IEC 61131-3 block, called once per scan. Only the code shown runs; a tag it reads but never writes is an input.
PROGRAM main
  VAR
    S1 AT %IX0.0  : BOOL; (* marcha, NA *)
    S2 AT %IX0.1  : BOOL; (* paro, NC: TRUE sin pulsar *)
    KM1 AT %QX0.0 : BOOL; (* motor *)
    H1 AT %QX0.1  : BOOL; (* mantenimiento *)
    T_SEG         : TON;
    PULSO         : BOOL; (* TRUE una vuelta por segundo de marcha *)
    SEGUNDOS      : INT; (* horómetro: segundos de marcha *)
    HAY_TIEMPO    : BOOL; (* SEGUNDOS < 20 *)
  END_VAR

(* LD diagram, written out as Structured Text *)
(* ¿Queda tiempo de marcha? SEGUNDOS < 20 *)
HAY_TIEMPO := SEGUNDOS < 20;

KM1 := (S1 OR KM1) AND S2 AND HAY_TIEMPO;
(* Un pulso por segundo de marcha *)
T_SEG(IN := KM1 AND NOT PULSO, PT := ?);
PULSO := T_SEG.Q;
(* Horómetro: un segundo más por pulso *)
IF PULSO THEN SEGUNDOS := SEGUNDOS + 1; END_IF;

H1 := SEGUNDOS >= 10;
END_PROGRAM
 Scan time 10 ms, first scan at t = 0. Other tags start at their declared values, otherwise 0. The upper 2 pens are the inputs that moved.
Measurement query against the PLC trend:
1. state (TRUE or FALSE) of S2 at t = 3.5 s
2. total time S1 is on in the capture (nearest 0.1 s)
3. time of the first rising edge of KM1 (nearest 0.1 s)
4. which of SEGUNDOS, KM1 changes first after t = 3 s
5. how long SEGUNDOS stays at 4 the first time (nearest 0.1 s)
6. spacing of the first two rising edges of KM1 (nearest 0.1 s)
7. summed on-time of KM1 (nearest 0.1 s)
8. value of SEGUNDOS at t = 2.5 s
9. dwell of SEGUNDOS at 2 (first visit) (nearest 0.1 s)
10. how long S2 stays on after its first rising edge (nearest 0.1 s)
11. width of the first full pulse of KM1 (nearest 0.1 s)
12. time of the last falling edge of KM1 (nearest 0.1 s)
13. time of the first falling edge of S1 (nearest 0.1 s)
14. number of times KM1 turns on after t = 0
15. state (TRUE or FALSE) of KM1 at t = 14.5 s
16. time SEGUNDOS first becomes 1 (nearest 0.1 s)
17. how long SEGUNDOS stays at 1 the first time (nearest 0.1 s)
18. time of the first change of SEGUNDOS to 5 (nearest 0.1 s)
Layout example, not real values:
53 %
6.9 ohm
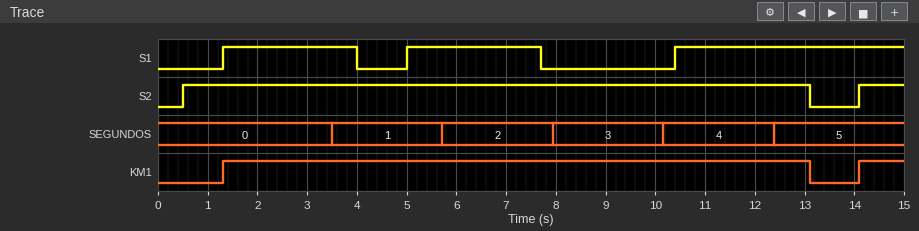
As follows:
TRUE
10.0 s
1.3 s
SEGUNDOS
2.2 s
12.8 s
12.7 s
0
2.2 s
12.6 s
11.8 s
13.1 s
4.0 s
2
TRUE
3.5 s
2.2 s
12.4 s
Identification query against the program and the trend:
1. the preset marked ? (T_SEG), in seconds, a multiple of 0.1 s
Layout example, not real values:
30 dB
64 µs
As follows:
2.2 s
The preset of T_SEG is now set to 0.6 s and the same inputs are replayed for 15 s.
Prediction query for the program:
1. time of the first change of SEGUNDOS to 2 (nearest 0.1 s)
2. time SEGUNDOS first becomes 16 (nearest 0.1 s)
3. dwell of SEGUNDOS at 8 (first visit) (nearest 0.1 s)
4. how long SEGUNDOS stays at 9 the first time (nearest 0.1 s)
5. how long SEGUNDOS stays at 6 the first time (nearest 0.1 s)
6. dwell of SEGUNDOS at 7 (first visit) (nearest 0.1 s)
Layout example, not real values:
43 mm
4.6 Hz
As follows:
2.5 s
11.2 s
0.6 s
0.6 s
0.6 s
0.6 s
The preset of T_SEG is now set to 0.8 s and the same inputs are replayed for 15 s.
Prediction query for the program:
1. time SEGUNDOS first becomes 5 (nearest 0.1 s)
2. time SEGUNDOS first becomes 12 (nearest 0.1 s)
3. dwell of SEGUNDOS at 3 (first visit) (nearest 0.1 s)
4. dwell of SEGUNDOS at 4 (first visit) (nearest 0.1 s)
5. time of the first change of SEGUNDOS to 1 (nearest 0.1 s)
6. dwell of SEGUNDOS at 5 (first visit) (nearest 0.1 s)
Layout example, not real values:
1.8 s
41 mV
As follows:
5.4 s
11.1 s
0.8 s
0.8 s
2.1 s
0.8 s
